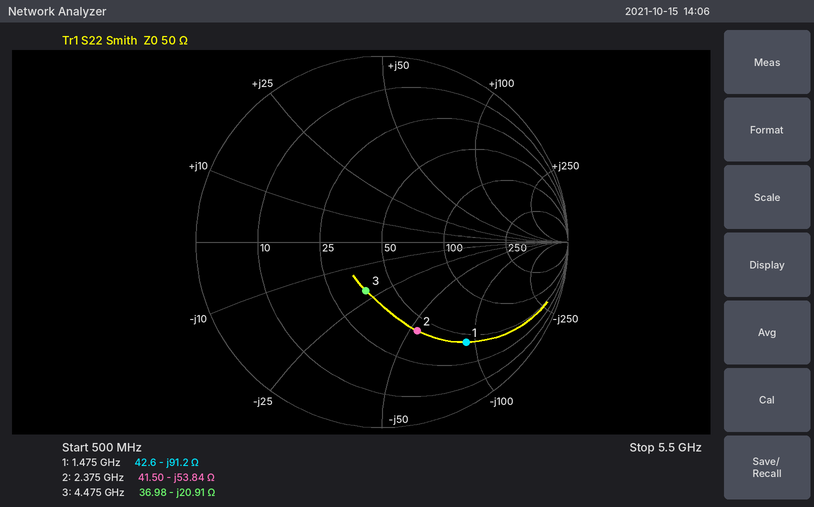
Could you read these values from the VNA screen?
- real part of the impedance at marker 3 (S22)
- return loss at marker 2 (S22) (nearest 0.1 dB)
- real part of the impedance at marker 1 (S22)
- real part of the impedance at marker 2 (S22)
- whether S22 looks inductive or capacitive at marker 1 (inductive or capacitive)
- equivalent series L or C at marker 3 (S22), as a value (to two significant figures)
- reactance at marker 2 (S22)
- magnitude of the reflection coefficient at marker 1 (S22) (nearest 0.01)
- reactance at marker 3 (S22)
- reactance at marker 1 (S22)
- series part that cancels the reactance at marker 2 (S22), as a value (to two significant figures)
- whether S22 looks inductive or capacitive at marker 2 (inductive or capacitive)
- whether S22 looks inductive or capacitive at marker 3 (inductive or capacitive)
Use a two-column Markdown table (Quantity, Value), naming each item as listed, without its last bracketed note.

| Quantity | Value |
|---|---|
| real part of the impedance at marker 3 | 36.98 Ω |
| return loss at marker 2 (S22) | 5.8 dB |
| real part of the impedance at marker 1 | 42.6 Ω |
| real part of the impedance at marker 2 | 41.50 Ω |
| whether S22 looks inductive or capacitive at marker 1 | capacitive |
| equivalent series L or C at marker 3 (S22), as a value | 1.7 pF |
| reactance at marker 2 | -53.84 Ω |
| magnitude of the reflection coefficient at marker 1 (S22) | 0.70 |
| reactance at marker 3 | -20.91 Ω |
| reactance at marker 1 | -91.2 Ω |
| series part that cancels the reactance at marker 2 (S22), as a value | 3.6 nH |
| whether S22 looks inductive or capacitive at marker 2 | capacitive |
| whether S22 looks inductive or capacitive at marker 3 | capacitive |
